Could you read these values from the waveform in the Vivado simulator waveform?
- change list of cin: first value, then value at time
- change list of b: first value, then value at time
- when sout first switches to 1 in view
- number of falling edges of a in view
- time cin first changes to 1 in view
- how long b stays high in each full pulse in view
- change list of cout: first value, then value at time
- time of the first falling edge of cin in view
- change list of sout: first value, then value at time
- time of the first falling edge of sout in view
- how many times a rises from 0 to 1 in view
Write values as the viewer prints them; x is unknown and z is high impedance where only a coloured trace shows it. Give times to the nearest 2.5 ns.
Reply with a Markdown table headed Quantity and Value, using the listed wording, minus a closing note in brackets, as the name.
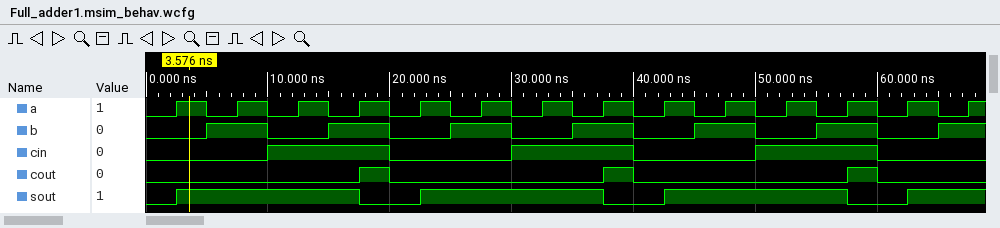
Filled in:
| Quantity | Value |
|---|---|
| change list of cin: first value, then value at time | 0, 1 at 10 ns, 0 at 20 ns, 1 at 30 ns, 0 at 40 ns, 1 at 50 ns, 0 at 60 ns |
| change list of b: first value, then value at time | 0, 1 at 5 ns, 0 at 10 ns, 1 at 15 ns, 0 at 20 ns, 1 at 25 ns, 0 at 30 ns, 1 at 35 ns, 0 at 40 ns, 1 at 45 ns, 0 at 50 ns, 1 at 55 ns, 0 at 60 ns, 1 at 65 ns |
| when sout first switches to 1 in view | 2.5 ns |
| number of falling edges of a in view | 13 |
| time cin first changes to 1 in view | 10 ns |
| how long b stays high in each full pulse in view | 5 ns, 5 ns, 5 ns, 5 ns, 5 ns, 5 ns |
| change list of cout: first value, then value at time | 0, 1 at 17.5 ns, 0 at 20 ns, 1 at 37.5 ns, 0 at 40 ns, 1 at 57.5 ns, 0 at 60 ns |
| time of the first falling edge of cin in view | 20 ns |
| change list of sout: first value, then value at time | 0, 1 at 2.5 ns, 0 at 17.5 ns, 1 at 22.5 ns, 0 at 37.5 ns, 1 at 42.5 ns, 0 at 57.5 ns, 1 at 62.5 ns |
| time of the first falling edge of sout in view | 17.5 ns |
| how many times a rises from 0 to 1 in view | 14 |
